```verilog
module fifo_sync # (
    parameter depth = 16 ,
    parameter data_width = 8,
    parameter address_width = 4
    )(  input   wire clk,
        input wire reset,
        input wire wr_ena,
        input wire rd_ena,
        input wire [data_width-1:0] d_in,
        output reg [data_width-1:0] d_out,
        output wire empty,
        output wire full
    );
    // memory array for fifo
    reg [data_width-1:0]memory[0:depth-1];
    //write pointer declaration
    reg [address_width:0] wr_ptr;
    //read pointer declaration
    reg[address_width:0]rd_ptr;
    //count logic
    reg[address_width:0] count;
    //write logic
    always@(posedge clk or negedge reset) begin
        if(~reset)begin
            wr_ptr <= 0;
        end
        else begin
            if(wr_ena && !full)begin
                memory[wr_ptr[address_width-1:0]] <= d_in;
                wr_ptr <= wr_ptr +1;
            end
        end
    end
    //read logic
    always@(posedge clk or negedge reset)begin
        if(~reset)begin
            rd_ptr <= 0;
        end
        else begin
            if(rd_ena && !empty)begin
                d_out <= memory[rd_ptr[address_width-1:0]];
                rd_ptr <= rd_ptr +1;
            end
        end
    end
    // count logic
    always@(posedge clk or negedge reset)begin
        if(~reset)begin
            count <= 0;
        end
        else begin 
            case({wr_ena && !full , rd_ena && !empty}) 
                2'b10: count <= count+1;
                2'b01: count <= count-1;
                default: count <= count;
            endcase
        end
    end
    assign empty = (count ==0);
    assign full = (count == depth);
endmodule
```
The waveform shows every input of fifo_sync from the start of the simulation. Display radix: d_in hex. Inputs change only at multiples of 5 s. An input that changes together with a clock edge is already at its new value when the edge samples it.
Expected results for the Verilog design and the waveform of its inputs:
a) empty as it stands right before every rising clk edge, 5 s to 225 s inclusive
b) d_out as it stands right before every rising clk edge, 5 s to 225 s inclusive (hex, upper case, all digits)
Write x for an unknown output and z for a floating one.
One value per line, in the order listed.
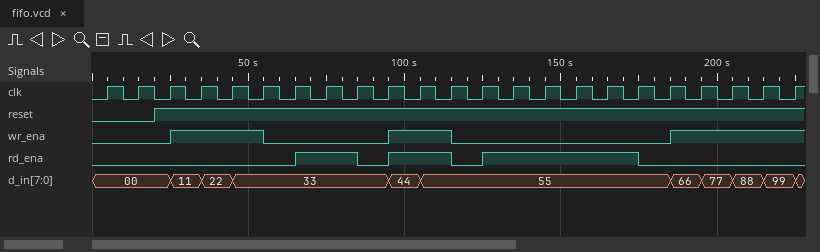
1 1 1 0 0 0 0 0 0 0 0 0 0 1 1 1 1 1 1 0 0 0 0
x, x, x, x, x, x, x, 11, 22, 22, 33, 44, 44, 55, 55, 55, 55, 55, 55, 55, 55, 55, 55
